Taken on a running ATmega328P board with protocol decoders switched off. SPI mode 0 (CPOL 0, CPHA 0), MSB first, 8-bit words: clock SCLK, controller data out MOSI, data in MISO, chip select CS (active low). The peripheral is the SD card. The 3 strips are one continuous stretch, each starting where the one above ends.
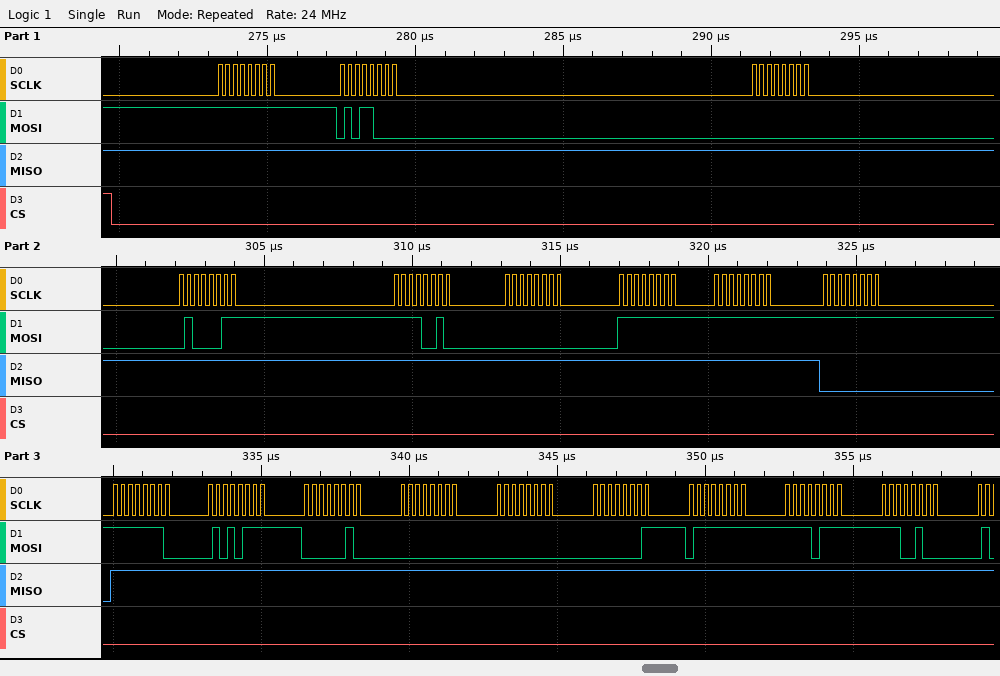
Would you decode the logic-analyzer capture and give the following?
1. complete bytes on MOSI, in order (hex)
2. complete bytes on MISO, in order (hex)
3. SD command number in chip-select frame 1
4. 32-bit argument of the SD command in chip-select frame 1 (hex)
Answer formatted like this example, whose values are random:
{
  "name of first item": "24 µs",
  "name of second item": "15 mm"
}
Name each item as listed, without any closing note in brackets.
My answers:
{
  "complete bytes on MOSI, in order": "0xFF 0x58 0x00 0x43 0xF2 0x00 0xFF 0xFF 0xFF 0xFE 0x57 0x02 0x00 0x00 0x01 0x7F 0xF7 0xE4",
  "complete bytes on MISO, in order": "0xFF 0xFF 0xFF 0xFF 0xFF 0xFF 0xFF 0xFF 0x00 0xFF 0xFF 0xFF 0xFF 0xFF 0xFF 0xFF 0xFF 0xFF",
  "SD command number in chip-select frame 1": "CMD24",
  "32-bit argument of the SD command in chip-select frame 1": "0x0043F200"
}
